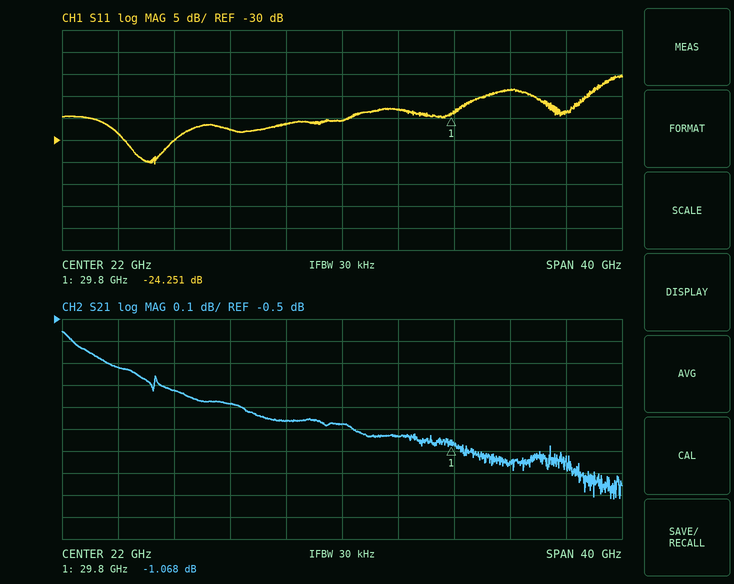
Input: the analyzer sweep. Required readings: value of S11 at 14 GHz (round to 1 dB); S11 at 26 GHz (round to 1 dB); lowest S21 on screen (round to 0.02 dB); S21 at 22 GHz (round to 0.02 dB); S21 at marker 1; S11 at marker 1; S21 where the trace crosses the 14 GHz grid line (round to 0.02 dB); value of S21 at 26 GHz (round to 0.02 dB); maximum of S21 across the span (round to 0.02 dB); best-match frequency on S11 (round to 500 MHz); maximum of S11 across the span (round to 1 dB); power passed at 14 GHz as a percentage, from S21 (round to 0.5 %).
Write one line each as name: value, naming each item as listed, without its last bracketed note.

value of S11 at 14 GHz: -28 dB
S11 at 26 GHz: -23 dB
lowest S21 on screen: -1.32 dB
S21 at 22 GHz: -0.98 dB
S21 at marker 1: -1.068 dB
S11 at marker 1: -24.251 dB
S21 where the trace crosses the 14 GHz grid line: -0.88 dB
value of S21 at 26 GHz: -1.04 dB
maximum of S21 across the span: -0.56 dB
best-match frequency on S11: 8.5 GHz
maximum of S11 across the span: -15 dB
power passed at 14 GHz as a percentage, from S21: 81.5 %
